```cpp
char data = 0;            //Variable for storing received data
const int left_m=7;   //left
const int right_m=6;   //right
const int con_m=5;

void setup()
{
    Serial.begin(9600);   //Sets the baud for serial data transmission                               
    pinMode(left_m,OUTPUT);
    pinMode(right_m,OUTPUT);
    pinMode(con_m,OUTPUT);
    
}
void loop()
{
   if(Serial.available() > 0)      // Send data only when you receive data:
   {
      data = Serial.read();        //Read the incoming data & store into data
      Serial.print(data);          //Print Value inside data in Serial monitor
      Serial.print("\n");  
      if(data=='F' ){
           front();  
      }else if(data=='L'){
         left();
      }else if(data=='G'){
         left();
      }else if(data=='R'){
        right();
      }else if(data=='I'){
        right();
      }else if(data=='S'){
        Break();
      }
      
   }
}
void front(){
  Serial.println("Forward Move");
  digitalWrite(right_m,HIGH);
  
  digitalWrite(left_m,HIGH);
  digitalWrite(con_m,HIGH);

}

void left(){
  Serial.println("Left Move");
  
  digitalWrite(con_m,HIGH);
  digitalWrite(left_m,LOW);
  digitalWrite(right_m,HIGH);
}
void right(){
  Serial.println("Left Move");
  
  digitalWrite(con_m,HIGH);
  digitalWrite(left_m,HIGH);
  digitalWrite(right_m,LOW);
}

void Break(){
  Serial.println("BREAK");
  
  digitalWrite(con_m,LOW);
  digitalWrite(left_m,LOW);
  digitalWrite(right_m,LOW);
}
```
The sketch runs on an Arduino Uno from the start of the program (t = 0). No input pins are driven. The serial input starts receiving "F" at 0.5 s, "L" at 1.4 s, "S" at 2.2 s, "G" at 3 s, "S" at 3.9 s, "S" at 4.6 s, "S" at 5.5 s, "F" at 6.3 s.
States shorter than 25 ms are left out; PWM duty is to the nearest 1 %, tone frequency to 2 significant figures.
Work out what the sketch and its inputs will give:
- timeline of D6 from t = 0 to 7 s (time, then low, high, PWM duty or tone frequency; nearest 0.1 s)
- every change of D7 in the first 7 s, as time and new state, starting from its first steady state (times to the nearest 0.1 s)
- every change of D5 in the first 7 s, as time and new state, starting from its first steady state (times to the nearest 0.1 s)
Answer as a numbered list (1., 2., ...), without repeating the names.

1. 0 s low; 0.5 s high; 2.2 s low; 3 s high; 3.9 s low; 6.3 s high
2. 0 s low; 0.5 s high; 1.4 s low; 6.3 s high
3. 0 s low; 0.5 s high; 2.2 s low; 3 s high; 3.9 s low; 6.3 s high
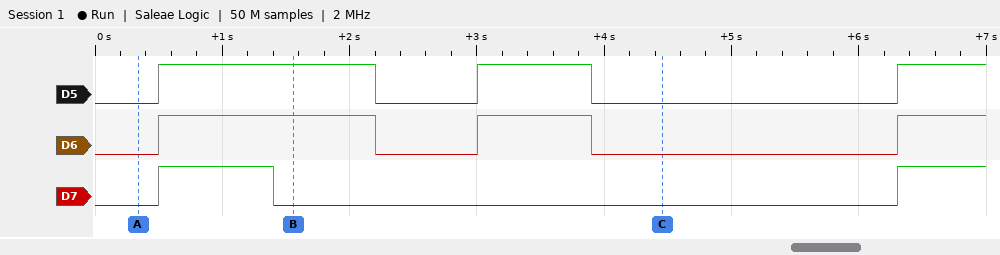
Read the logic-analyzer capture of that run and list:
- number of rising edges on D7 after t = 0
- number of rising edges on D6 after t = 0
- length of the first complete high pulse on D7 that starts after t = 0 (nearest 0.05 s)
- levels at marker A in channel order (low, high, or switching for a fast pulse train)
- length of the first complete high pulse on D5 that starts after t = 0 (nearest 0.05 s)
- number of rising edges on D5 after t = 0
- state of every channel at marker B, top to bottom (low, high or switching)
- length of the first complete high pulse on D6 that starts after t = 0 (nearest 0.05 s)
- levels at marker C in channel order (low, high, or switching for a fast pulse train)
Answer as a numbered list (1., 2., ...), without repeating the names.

1. 2
2. 3
3. 0.90 s
4. D5 low, D6 low, D7 low
5. 1.70 s
6. 3
7. D5 high, D6 high, D7 low
8. 1.70 s
9. D5 low, D6 low, D7 low
